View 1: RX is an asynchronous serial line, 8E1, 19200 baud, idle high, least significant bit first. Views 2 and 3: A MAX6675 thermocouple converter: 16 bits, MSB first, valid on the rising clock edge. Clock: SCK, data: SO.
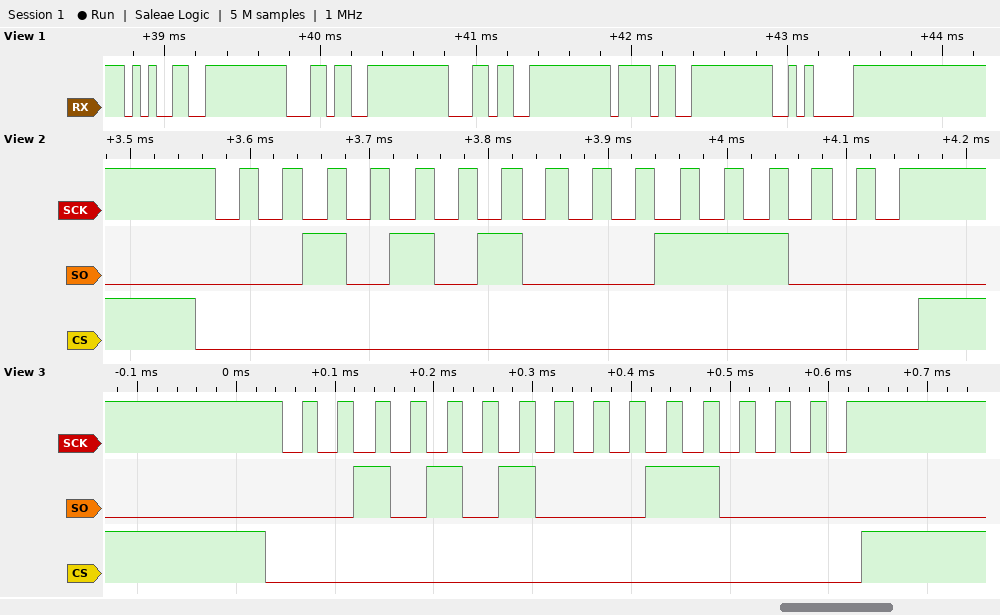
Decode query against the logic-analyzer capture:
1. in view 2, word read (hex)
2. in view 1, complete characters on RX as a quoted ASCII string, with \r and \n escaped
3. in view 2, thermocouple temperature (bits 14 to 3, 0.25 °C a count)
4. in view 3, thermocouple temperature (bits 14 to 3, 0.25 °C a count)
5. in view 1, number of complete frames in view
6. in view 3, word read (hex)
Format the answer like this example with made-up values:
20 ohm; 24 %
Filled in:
0x2A38; "ello\n"; 337.75 °C; 337.50 °C; 5; 0x2A30
